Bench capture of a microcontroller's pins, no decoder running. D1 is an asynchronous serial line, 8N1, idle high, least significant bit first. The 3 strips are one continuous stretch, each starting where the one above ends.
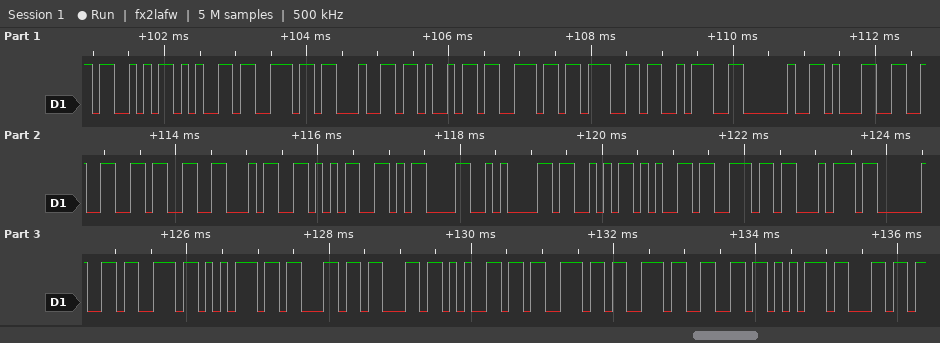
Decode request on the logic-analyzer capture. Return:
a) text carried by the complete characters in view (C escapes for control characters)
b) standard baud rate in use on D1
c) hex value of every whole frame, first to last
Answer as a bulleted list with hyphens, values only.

- "Sending: 12345\r\nSent successful"
- 9600 baud
- 53 65 6E 64 69 6E 67 3A 20 31 32 33 34 35 0D 0A 53 65 6E 74 20 73 75 63 63 65 73 73 66 75 6C
